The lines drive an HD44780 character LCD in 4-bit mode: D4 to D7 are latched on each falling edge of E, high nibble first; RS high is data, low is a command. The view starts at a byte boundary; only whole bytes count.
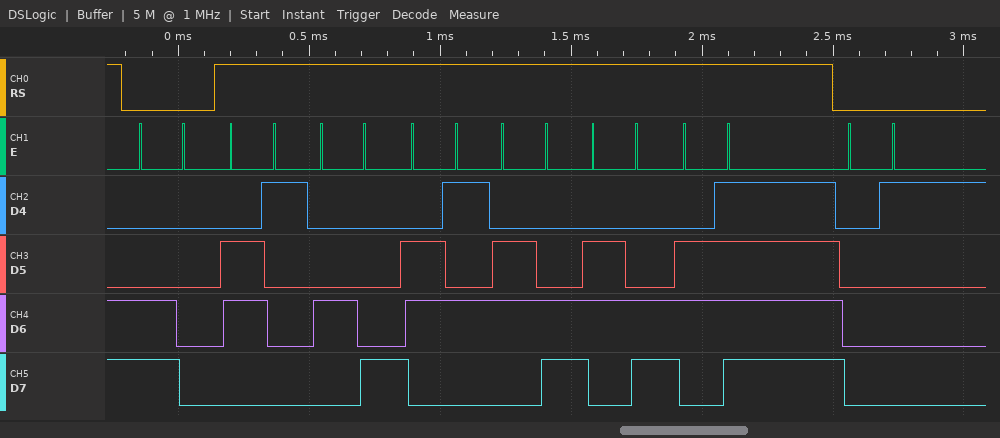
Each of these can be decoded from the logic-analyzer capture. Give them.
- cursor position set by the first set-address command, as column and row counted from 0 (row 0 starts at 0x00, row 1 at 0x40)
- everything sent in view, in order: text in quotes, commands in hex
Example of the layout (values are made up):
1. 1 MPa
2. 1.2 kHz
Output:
1. column 0, row 1
2. 0xC0 "aHello" 0x01
